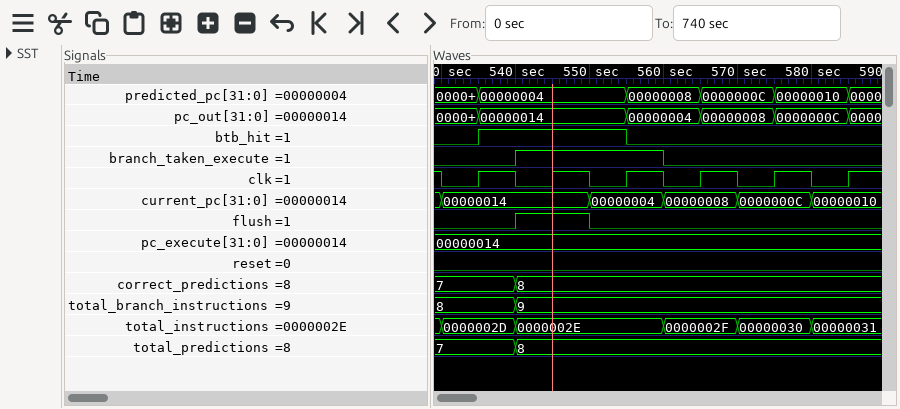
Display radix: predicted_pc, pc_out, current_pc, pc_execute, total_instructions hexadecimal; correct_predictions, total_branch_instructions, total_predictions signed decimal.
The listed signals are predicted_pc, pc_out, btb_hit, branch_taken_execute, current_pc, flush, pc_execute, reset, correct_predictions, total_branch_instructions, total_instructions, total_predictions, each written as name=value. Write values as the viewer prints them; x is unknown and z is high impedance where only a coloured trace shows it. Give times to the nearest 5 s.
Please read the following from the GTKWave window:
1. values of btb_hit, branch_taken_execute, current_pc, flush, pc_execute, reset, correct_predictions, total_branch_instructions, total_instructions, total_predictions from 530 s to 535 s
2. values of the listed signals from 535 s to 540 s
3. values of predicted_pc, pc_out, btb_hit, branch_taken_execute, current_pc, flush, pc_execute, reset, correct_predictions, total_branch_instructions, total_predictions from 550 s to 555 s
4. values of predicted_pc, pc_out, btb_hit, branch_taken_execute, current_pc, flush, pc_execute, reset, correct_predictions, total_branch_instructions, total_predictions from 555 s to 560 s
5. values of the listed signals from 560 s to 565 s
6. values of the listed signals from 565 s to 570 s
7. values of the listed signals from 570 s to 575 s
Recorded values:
btb_hit=0, branch_taken_execute=0, current_pc=00000014, flush=0, pc_execute=00000014, reset=0, correct_predictions=7, total_branch_instructions=8, total_instructions=0000002D, total_predictions=7
predicted_pc=00000004, pc_out=00000014, btb_hit=1, branch_taken_execute=0, current_pc=00000014, flush=0, pc_execute=00000014, reset=0, correct_predictions=7, total_branch_instructions=8, total_instructions=0000002D, total_predictions=7
predicted_pc=00000004, pc_out=00000014, btb_hit=1, branch_taken_execute=1, current_pc=00000004, flush=0, pc_execute=00000014, reset=0, correct_predictions=8, total_branch_instructions=9, total_predictions=8
predicted_pc=00000008, pc_out=00000004, btb_hit=0, branch_taken_execute=1, current_pc=00000004, flush=0, pc_execute=00000014, reset=0, correct_predictions=8, total_branch_instructions=9, total_predictions=8
predicted_pc=00000008, pc_out=00000004, btb_hit=0, branch_taken_execute=0, current_pc=00000008, flush=0, pc_execute=00000014, reset=0, correct_predictions=8, total_branch_instructions=9, total_instructions=0000002F, total_predictions=8
predicted_pc=0000000C, pc_out=00000008, btb_hit=0, branch_taken_execute=0, current_pc=00000008, flush=0, pc_execute=00000014, reset=0, correct_predictions=8, total_branch_instructions=9, total_instructions=0000002F, total_predictions=8
predicted_pc=0000000C, pc_out=00000008, btb_hit=0, branch_taken_execute=0, current_pc=0000000C, flush=0, pc_execute=00000014, reset=0, correct_predictions=8, total_branch_instructions=9, total_instructions=00000030, total_predictions=8
